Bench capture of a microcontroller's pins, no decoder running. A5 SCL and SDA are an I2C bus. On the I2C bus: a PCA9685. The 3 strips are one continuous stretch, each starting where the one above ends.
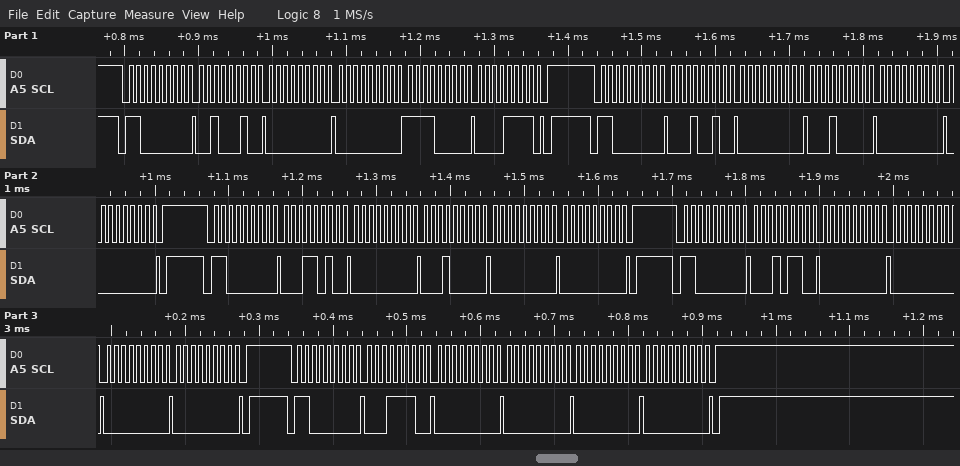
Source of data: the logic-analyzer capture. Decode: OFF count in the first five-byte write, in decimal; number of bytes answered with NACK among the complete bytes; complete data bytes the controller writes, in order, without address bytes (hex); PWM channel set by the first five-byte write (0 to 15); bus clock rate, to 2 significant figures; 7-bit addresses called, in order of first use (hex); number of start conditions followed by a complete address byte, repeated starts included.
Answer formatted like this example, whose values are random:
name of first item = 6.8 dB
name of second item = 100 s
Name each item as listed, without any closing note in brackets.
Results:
OFF count in the first five-byte write, in decimal = 4080
number of bytes answered with NACK among the complete bytes = 0
complete data bytes the controller writes, in order, without address bytes = 22 00 00 F0 0F 12 00 10 00 00 1A 00 10 00 00 16 00 00 00 00 1E 00 00 00 00
PWM channel set by the first five-byte write = 7
bus clock rate, to 2 significant figures = 100 kHz
7-bit addresses called, in order of first use = 0x60
number of start conditions followed by a complete address byte, repeated starts included = 5
